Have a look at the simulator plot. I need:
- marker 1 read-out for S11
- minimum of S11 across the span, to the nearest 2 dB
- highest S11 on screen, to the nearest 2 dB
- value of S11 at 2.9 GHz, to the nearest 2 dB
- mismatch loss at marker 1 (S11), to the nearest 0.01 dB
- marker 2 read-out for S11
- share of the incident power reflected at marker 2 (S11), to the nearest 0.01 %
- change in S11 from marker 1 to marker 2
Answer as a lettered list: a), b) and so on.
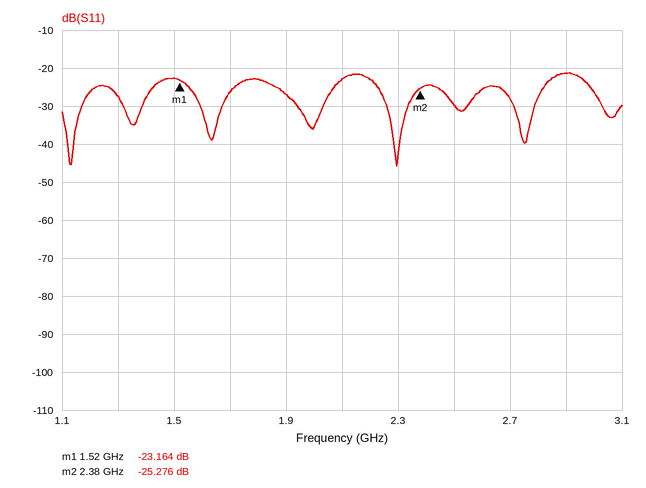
a) -23.164 dB
b) -46 dB
c) -22 dB
d) -22 dB
e) 0.02 dB
f) -25.276 dB
g) 0.30 %
h) -2.112 dB
